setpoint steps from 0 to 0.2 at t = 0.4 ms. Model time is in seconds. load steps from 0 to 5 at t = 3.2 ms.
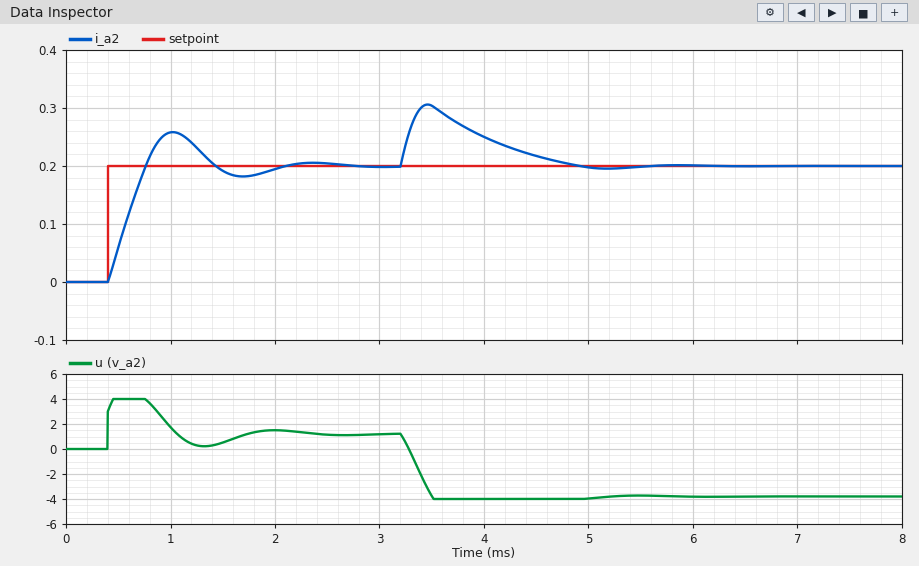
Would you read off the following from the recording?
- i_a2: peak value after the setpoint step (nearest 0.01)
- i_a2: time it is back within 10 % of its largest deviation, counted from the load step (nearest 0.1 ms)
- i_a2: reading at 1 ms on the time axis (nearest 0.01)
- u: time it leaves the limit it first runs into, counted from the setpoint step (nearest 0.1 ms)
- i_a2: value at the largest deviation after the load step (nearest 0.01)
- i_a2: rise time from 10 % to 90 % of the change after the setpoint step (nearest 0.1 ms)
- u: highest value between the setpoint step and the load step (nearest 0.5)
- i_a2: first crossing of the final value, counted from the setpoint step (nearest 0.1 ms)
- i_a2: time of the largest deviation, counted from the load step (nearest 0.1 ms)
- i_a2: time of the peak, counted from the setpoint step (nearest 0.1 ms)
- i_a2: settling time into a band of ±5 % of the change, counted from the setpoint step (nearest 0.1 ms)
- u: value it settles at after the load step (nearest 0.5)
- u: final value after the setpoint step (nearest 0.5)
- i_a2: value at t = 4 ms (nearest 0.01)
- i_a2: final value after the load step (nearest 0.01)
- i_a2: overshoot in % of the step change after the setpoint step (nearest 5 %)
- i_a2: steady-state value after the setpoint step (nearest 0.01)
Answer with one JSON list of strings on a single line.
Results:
["0.26", "1.4 ms", "0.26", "0.4 ms", "0.31", "0.3 ms", "4.0", "0.4 ms", "0.3 ms", "0.6 ms", "1.5 ms", "-4.0", "1.0", "0.25", "0.20", "30 %", "0.20"]
